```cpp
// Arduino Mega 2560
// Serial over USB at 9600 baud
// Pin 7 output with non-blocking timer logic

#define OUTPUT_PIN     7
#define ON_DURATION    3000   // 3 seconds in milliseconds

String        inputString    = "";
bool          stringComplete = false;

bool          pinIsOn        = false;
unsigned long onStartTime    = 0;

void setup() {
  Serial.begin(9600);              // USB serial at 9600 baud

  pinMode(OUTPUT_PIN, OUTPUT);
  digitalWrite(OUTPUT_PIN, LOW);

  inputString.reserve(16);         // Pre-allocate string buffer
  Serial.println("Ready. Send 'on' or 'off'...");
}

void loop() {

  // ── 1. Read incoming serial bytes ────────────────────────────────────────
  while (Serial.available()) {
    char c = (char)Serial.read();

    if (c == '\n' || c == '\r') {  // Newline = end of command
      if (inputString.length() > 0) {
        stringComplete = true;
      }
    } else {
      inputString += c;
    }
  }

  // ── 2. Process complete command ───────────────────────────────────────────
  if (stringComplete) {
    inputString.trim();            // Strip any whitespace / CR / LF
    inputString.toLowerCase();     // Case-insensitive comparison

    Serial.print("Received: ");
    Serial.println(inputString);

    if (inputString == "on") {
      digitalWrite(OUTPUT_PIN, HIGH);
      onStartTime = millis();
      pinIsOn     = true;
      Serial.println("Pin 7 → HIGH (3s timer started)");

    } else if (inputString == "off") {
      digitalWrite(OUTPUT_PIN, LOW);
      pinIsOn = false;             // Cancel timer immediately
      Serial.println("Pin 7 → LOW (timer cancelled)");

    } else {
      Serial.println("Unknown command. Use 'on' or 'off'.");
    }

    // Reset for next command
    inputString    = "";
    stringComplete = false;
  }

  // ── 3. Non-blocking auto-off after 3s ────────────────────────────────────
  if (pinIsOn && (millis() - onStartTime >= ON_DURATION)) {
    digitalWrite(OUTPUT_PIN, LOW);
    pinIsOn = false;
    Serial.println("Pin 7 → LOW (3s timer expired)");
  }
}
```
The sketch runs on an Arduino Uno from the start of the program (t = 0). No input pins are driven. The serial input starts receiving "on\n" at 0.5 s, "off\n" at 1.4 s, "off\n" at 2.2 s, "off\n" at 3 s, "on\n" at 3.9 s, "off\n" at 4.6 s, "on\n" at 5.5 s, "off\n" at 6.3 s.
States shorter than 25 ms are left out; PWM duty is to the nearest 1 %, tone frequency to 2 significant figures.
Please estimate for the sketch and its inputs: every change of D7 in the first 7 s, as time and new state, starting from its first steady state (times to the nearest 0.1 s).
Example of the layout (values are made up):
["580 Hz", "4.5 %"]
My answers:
["0 s low; 0.5 s high; 1.4 s low; 3.9 s high; 4.6 s low; 5.5 s high; 6.3 s low"]
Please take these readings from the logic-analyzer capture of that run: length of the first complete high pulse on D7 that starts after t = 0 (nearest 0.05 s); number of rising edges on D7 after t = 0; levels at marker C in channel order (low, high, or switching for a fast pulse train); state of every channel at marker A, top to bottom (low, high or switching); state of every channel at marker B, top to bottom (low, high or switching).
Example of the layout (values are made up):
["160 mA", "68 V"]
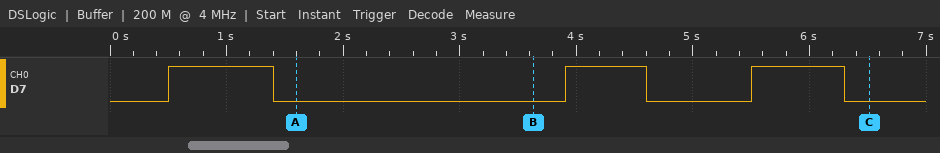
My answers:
["0.90 s", "3", "D7 low", "D7 low", "D7 low"]
